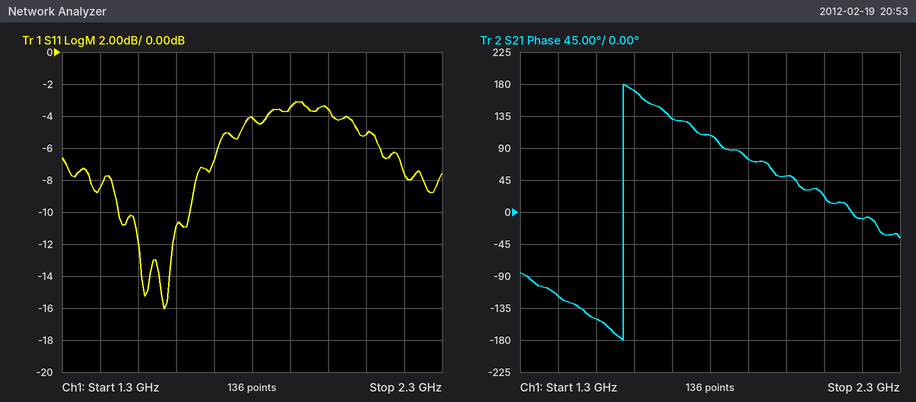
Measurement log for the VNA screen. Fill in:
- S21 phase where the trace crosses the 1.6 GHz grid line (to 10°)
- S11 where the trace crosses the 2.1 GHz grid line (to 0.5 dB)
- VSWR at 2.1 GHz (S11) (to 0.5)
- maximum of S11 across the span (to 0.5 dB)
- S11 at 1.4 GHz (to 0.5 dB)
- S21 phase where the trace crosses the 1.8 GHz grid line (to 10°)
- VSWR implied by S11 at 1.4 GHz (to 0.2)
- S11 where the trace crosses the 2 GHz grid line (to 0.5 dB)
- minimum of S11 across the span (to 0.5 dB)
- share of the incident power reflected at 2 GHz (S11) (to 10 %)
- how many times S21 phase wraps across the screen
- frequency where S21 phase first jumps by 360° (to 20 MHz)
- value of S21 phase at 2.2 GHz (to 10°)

170°
-5.0 dB
3.5
-3.0 dB
-8.5 dB
110°
2.2
-3.5 dB
-16.0 dB
40 %
1
1.58 GHz
-10°
